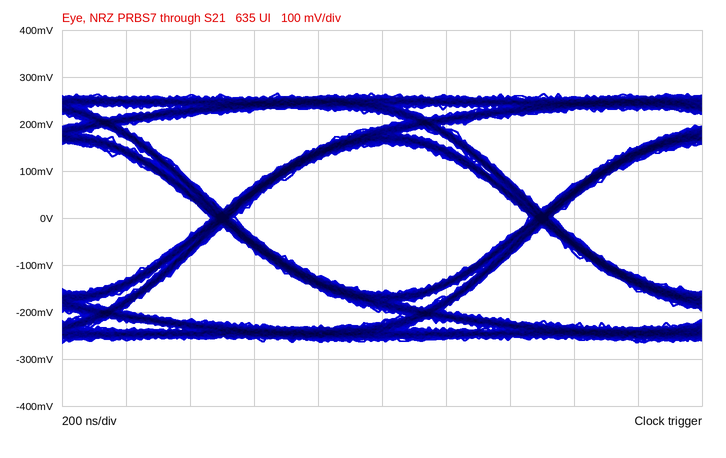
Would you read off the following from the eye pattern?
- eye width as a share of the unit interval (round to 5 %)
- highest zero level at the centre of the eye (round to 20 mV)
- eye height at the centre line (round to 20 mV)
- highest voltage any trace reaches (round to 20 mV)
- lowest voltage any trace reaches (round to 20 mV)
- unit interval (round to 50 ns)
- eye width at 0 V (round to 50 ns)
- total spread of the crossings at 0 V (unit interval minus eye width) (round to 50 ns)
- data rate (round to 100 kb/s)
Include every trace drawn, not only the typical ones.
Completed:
90 %
-160 mV
320 mV
260 mV
-260 mV
1.00 µs
900 ns
100 ns
1.0 Mb/s
